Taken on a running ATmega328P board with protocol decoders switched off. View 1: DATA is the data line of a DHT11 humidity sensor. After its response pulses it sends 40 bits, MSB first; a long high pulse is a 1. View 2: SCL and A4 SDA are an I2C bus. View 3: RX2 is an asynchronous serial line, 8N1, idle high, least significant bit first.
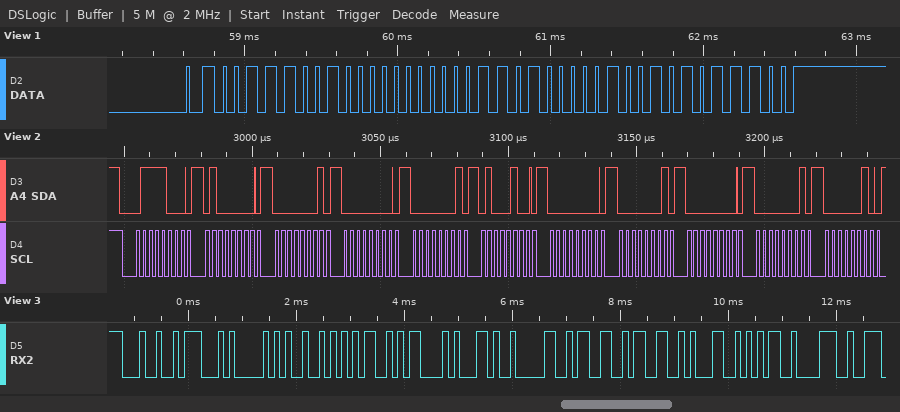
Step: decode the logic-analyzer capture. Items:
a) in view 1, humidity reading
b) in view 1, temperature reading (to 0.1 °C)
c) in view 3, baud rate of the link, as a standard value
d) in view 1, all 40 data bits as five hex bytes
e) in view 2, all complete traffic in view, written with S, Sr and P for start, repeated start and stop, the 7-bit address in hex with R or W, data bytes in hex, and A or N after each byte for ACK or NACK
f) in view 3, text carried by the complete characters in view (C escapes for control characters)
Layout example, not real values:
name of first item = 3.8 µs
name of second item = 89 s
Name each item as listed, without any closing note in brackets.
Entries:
in view 1, humidity reading = 57 %
in view 1, temperature reading = 26.9 °C
in view 3, baud rate of the link, as a standard value = 9600 baud
in view 1, all 40 data bits as five hex bytes = 39 00 1A 09 5C
in view 2, all complete traffic in view, written with S, Sr and P for start, repeated start and stop, the 7-bit address in hex with R or W, data bytes in hex, and A or N after each byte for ACK or NACK = S 3CW A 40 A 01 A 00 A 01 A 44 A 00 A 01 A 00 A 01 A 02 A
in view 3, text carried by the complete characters in view = "$GPRMC,033158"
